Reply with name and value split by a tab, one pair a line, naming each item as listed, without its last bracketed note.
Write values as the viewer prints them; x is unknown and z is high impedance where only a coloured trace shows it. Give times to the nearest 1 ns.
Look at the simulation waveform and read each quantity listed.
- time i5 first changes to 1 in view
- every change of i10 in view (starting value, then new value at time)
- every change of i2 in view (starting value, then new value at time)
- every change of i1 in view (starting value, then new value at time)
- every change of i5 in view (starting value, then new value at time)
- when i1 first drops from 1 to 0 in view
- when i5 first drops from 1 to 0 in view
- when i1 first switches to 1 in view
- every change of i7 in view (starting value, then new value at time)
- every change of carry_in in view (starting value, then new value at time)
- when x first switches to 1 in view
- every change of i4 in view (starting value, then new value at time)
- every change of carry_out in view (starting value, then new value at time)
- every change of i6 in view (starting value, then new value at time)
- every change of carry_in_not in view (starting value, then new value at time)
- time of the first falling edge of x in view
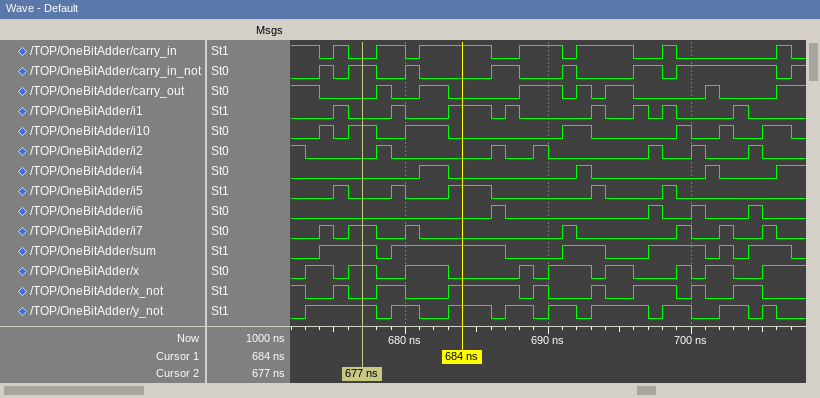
time i5 first changes to 1 in view	675 ns
every change of i10 in view	0, 1 at 674 ns, 0 at 675 ns, 1 at 676 ns, 0 at 678 ns, 1 at 680 ns, 0 at 683 ns, 1 at 691 ns, 0 at 693 ns, 1 at 699 ns, 0 at 700 ns, 1 at 702 ns, 0 at 703 ns, 1 at 705 ns, 0 at 707 ns
every change of i2 in view	1, 0 at 673 ns, 1 at 678 ns, 0 at 679 ns, 1 at 686 ns, 0 at 687 ns, 1 at 689 ns, 0 at 690 ns, 1 at 697 ns, 0 at 698 ns, 1 at 700 ns, 0 at 701 ns, 1 at 704 ns, 0 at 705 ns
every change of i1 in view	0, 1 at 675 ns, 0 at 676 ns, 1 at 679 ns, 0 at 680 ns, 1 at 683 ns, 0 at 686 ns, 1 at 687 ns, 0 at 688 ns, 1 at 693 ns, 0 at 694 ns, 1 at 696 ns, 0 at 697 ns, 1 at 698 ns, 0 at 699 ns, 1 at 703 ns, 0 at 704 ns
every change of i5 in view	0, 1 at 675 ns, 0 at 676 ns, 1 at 679 ns, 0 at 680 ns, 1 at 683 ns, 0 at 686 ns, 1 at 693 ns, 0 at 694 ns, 1 at 698 ns, 0 at 699 ns
when i1 first drops from 1 to 0 in view	676 ns
when i5 first drops from 1 to 0 in view	676 ns
when i1 first switches to 1 in view	675 ns
every change of i7 in view	0, 1 at 674 ns, 0 at 675 ns, 1 at 676 ns, 0 at 678 ns, 1 at 680 ns, 0 at 681 ns, 1 at 691 ns, 0 at 692 ns, 1 at 699 ns, 0 at 700 ns, 1 at 702 ns, 0 at 703 ns, 1 at 705 ns, 0 at 706 ns
every change of carry_in in view	1, 0 at 674 ns, 1 at 675 ns, 0 at 676 ns, 1 at 678 ns, 0 at 680 ns, 1 at 681 ns, 0 at 686 ns, 1 at 688 ns, 0 at 691 ns, 1 at 692 ns, 0 at 696 ns, 1 at 698 ns, 0 at 699 ns, 1 at 706 ns, 0 at 707 ns
when x first switches to 1 in view	673 ns
every change of i4 in view	0, 1 at 681 ns, 0 at 683 ns, 1 at 692 ns, 0 at 693 ns, 1 at 701 ns, 0 at 702 ns, 1 at 706 ns
every change of carry_out in view	1, 0 at 674 ns, 1 at 678 ns, 0 at 679 ns, 1 at 681 ns, 0 at 683 ns, 1 at 688 ns, 0 at 691 ns, 1 at 692 ns, 0 at 693 ns, 1 at 694 ns, 0 at 696 ns, 1 at 701 ns, 0 at 702 ns, 1 at 706 ns
every change of i6 in view	0, 1 at 686 ns, 0 at 687 ns, 1 at 697 ns, 0 at 698 ns, 1 at 700 ns, 0 at 701 ns, 1 at 704 ns, 0 at 705 ns
every change of carry_in_not in view	0, 1 at 674 ns, 0 at 675 ns, 1 at 676 ns, 0 at 678 ns, 1 at 680 ns, 0 at 681 ns, 1 at 686 ns, 0 at 688 ns, 1 at 691 ns, 0 at 692 ns, 1 at 696 ns, 0 at 698 ns, 1 at 699 ns, 0 at 706 ns, 1 at 707 ns
time of the first falling edge of x in view	675 ns
